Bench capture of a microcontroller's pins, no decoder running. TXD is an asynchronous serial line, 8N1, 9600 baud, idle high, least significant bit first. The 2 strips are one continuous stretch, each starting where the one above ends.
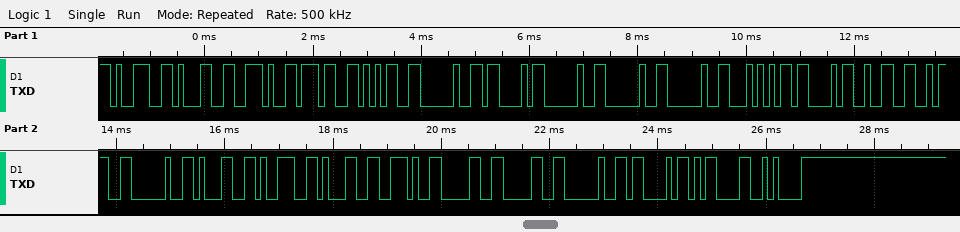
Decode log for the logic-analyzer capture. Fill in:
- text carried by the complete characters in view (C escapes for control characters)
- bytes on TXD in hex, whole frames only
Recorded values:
"91.75 C   TC2: 191.00 C\r\n"
0x39 0x31 0x2E 0x37 0x35 0x20 0x43 0x20 0x20 0x20 0x54 0x43 0x32 0x3A 0x20 0x31 0x39 0x31 0x2E 0x30 0x30 0x20 0x43 0x0D 0x0A
